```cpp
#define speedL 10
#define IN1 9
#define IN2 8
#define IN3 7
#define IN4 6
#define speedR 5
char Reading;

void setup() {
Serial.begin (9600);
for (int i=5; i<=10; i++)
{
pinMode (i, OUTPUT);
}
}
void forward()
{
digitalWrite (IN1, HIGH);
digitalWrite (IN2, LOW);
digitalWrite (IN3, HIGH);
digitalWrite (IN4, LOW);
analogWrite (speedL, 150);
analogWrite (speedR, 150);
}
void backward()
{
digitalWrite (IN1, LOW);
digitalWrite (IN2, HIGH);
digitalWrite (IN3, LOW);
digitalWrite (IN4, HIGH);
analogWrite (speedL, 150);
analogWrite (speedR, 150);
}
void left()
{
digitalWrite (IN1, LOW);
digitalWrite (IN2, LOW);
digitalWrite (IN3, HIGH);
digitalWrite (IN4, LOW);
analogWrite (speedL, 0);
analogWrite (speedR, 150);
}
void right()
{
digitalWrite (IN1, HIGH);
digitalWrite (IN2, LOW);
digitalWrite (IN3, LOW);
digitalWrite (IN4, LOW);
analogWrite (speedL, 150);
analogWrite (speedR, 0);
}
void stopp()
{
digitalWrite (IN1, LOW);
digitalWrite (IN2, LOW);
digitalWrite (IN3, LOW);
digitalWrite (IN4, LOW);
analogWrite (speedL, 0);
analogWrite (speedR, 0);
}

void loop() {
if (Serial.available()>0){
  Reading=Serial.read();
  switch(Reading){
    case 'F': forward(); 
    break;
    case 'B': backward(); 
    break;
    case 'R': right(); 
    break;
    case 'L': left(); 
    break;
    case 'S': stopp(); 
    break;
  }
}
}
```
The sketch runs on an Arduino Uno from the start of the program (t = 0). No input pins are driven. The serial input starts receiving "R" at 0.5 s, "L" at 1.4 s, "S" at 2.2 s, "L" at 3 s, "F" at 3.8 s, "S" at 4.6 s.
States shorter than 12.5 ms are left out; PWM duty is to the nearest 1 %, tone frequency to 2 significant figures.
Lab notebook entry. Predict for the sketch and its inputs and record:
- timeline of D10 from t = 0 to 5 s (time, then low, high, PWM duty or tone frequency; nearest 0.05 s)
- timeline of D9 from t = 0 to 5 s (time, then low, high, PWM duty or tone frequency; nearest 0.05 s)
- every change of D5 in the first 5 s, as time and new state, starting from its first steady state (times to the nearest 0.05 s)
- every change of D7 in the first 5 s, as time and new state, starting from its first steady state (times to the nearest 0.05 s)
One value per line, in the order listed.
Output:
0 s low; 0.5 s PWM 59 %; 1.4 s low; 3.8 s PWM 59 %; 4.6 s low
0 s low; 0.5 s high; 1.4 s low; 3.8 s high; 4.6 s low
0 s low; 1.4 s PWM 59 %; 2.2 s low; 3 s PWM 59 %; 4.6 s low
0 s low; 1.4 s high; 2.2 s low; 3 s high; 4.6 s low
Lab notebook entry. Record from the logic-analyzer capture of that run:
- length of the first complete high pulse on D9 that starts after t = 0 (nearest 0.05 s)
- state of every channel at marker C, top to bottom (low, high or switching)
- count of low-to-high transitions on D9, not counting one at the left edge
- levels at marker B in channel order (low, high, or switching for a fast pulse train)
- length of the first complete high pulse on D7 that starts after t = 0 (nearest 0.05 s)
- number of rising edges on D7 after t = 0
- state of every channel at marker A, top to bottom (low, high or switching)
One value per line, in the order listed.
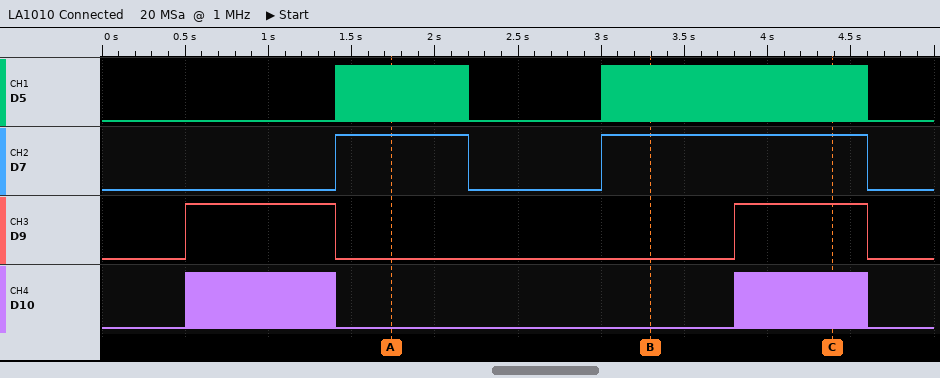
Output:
0.90 s
D5 switching, D7 high, D9 high, D10 switching
2
D5 switching, D7 high, D9 low, D10 low
0.80 s
2
D5 switching, D7 high, D9 low, D10 low
